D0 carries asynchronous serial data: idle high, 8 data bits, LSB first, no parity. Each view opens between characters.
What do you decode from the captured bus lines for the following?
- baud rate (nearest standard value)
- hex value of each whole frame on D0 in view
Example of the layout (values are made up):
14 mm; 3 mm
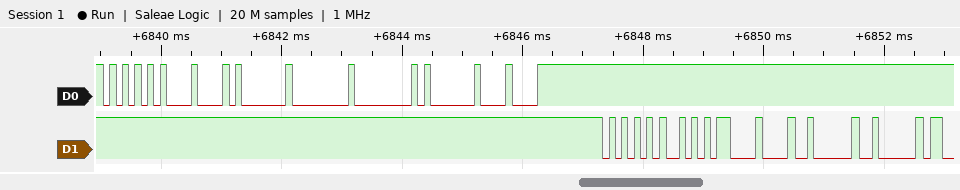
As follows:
9600 baud; 55, 08, 01, 00, 00, 01, 08
